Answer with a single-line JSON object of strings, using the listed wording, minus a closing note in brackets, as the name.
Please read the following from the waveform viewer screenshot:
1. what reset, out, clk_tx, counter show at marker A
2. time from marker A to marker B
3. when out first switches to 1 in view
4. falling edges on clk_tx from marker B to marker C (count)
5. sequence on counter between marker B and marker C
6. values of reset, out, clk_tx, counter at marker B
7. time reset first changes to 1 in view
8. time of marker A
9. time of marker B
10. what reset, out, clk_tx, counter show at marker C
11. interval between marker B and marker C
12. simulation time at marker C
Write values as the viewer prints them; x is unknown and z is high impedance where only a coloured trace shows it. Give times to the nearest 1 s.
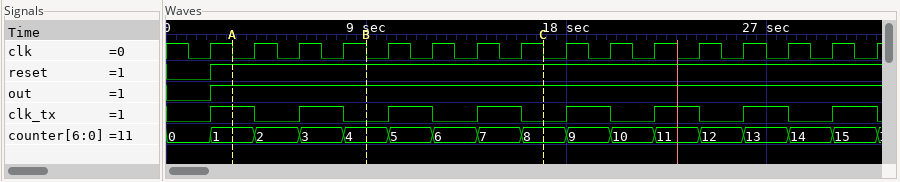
{"what reset, out, clk_tx, counter show at marker A": "reset=1, out=1, clk_tx=1, counter=1", "time from marker A to marker B": "6 s", "when out first switches to 1 in view": "2 s", "falling edges on clk_tx from marker B to marker C": "2", "sequence on counter between marker B and marker C": "4, 5, 6, 7, 8", "values of reset, out, clk_tx, counter at marker B": "reset=1, out=1, clk_tx=0, counter=4", "time reset first changes to 1 in view": "2 s", "time of marker A": "3 s", "time of marker B": "9 s", "what reset, out, clk_tx, counter show at marker C": "reset=1, out=1, clk_tx=0, counter=8", "interval between marker B and marker C": "8 s", "simulation time at marker C": "17 s"}
